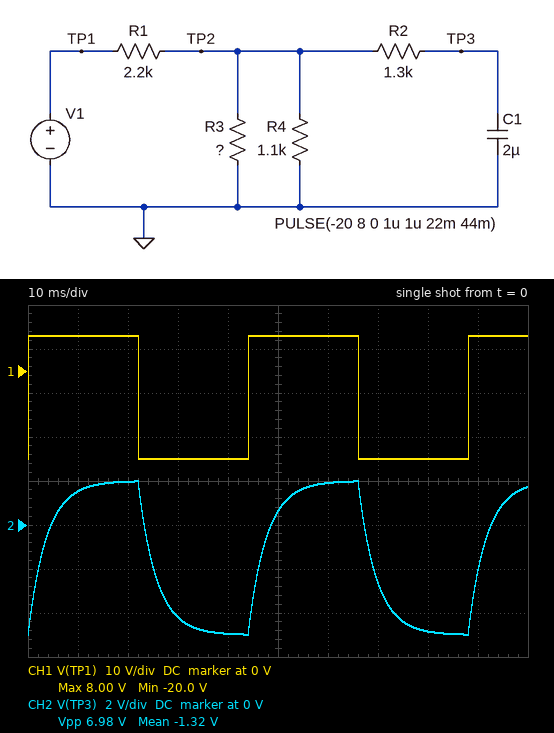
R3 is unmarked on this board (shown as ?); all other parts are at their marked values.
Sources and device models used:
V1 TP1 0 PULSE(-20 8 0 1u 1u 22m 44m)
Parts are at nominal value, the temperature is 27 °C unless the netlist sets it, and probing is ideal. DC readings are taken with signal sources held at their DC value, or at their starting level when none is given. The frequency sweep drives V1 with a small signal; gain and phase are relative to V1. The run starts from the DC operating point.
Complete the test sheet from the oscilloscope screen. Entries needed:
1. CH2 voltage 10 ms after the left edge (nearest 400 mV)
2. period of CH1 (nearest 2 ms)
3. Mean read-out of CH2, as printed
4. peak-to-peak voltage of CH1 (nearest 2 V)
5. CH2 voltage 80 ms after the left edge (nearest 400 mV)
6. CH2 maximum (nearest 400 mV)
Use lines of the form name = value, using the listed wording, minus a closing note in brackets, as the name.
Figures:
CH2 voltage 10 ms after the left edge = 1.6 V
period of CH1 = 44 ms
Mean read-out of CH2, as printed = -1.32 V
peak-to-peak voltage of CH1 = 28 V
CH2 voltage 80 ms after the left edge = -4.8 V
CH2 maximum = 2.0 V
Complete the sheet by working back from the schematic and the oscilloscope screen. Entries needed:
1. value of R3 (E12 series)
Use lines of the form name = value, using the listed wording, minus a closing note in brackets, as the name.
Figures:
value of R3 = 2.2 kΩ
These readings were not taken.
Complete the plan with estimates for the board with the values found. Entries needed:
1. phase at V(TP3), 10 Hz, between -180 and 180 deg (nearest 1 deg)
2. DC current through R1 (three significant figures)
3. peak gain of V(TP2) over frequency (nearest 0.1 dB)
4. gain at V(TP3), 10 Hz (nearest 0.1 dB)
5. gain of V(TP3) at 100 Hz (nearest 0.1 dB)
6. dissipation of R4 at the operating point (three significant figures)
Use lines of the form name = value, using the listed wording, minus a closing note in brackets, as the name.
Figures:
phase at V(TP3), 10 Hz, between -180 and 180 deg = -13 deg
DC current through R1 = 6.82 mA
peak gain of V(TP2) over frequency = -12.0 dB
gain at V(TP3), 10 Hz = -12.3 dB
gain of V(TP3) at 100 Hz = -20.1 dB
dissipation of R4 at the operating point = 22.7 mW
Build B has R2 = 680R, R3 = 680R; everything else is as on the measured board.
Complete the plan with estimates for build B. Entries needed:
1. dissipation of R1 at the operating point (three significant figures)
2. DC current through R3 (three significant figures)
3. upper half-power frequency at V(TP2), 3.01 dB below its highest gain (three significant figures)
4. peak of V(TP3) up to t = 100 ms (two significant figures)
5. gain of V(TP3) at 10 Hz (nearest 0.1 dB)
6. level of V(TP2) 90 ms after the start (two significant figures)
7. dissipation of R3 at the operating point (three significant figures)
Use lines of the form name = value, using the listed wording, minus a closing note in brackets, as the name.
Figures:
dissipation of R1 at the operating point = 128 mW
DC current through R3 = 4.72 mA
upper half-power frequency at V(TP2), 3.01 dB below its highest gain = 211 Hz
peak of V(TP3) up to t = 100 ms = 1.3 V
gain of V(TP3) at 10 Hz = -16.0 dB
level of V(TP2) 90 ms after the start = 700 mV
dissipation of R3 at the operating point = 15.1 mW
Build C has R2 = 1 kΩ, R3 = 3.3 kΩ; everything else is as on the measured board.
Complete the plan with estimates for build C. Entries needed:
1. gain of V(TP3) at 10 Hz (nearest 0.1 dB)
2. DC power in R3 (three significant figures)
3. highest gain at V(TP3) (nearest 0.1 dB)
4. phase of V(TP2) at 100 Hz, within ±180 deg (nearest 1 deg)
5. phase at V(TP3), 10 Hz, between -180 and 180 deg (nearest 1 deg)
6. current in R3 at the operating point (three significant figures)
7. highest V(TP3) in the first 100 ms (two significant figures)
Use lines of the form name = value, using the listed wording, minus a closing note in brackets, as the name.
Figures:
gain of V(TP3) at 10 Hz = -11.5 dB
DC power in R3 = 9.02 mW
highest gain at V(TP3) = -11.3 dB
phase of V(TP2) at 100 Hz, within ±180 deg = -12 deg
phase at V(TP3), 10 Hz, between -180 and 180 deg = -11 deg
current in R3 at the operating point = 1.65 mA
highest V(TP3) in the first 100 ms = 2.2 V
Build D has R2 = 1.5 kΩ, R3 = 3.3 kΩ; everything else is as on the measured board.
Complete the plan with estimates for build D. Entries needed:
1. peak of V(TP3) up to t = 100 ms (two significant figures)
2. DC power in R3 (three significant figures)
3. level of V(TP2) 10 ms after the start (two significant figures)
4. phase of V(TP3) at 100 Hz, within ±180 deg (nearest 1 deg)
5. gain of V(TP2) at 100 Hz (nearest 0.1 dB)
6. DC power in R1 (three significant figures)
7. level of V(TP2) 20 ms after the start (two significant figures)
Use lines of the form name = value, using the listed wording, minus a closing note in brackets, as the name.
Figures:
peak of V(TP3) up to t = 100 ms = 2.1 V
DC power in R3 = 9.02 mW
level of V(TP2) 10 ms after the start = 2.0 V
phase of V(TP3) at 100 Hz, within ±180 deg = -69 deg
gain of V(TP2) at 100 Hz = -13.7 dB
DC power in R1 = 96.2 mW
level of V(TP2) 20 ms after the start = 2.2 V
